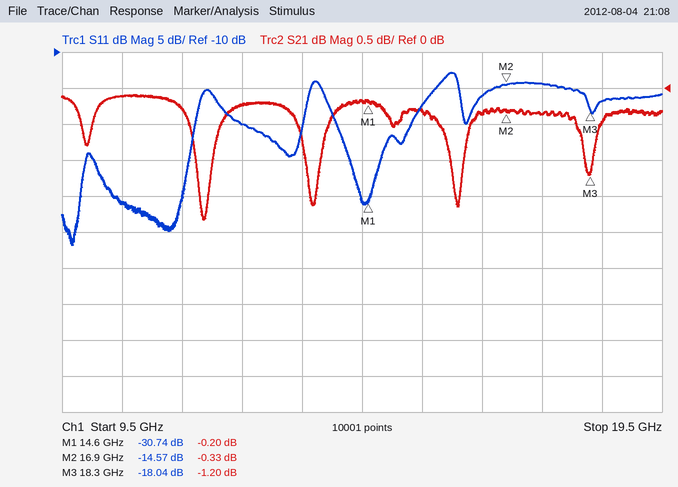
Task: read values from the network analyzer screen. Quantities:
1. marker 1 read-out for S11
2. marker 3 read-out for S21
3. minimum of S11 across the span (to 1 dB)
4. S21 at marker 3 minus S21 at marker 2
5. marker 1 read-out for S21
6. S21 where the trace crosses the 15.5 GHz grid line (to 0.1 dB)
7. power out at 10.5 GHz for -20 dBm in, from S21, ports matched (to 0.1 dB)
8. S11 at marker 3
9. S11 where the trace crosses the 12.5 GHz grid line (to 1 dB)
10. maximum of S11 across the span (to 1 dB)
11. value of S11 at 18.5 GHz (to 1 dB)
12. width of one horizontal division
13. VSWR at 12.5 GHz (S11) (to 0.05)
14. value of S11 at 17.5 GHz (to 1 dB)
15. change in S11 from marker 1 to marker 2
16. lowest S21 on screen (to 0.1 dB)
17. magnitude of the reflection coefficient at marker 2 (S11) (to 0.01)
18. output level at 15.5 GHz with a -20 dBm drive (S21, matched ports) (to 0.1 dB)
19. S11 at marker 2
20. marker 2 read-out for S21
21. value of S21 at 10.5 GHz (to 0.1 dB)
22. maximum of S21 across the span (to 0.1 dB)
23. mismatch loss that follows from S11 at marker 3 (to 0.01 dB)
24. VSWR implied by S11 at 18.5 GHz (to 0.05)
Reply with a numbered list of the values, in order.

1. -30.74 dB
2. -1.20 dB
3. -37 dB
4. -0.87 dB
5. -0.20 dB
6. -0.3 dB
7. -20.1 dBm
8. -18.04 dB
9. -20 dB
10. -13 dB
11. -17 dB
12. 1 GHz
13. 1.20
14. -14 dB
15. 16.17 dB
16. -1.8 dB
17. 0.19
18. -20.3 dBm
19. -14.57 dB
20. -0.33 dB
21. -0.1 dB
22. -0.1 dB
23. 0.07 dB
24. 1.35
